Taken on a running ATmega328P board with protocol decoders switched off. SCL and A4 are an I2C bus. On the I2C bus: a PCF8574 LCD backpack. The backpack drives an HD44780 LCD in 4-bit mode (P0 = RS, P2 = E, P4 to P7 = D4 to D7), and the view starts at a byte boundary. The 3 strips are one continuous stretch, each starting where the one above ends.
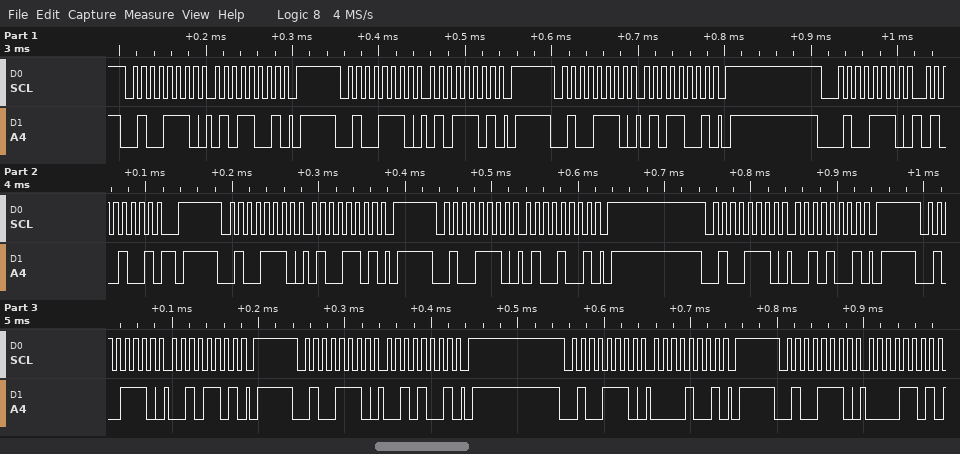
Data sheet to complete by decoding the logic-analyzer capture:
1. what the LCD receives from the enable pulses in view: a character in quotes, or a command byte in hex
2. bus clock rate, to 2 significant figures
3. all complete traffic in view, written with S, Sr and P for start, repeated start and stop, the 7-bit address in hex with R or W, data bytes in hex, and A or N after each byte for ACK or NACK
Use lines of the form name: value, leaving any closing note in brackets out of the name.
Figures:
what the LCD receives from the enable pulses in view: a character in quotes, or a command byte in hex: 'T'
bus clock rate, to 2 significant figures: 100 kHz
all complete traffic in view, written with S, Sr and P for start, repeated start and stop, the 7-bit address in hex with R or W, data bytes in hex, and A or N after each byte for ACK or NACK: S 27W A 59 A P S 27W A 5D A P S 27W A 59 A P S 27W A 49 A P S 27W A 4D A P S 27W A 49 A P S 27W A 29 A P S 27W A 2D A P S 27W A 29 A P S 27W A 09 A P S 27W A 0D A
